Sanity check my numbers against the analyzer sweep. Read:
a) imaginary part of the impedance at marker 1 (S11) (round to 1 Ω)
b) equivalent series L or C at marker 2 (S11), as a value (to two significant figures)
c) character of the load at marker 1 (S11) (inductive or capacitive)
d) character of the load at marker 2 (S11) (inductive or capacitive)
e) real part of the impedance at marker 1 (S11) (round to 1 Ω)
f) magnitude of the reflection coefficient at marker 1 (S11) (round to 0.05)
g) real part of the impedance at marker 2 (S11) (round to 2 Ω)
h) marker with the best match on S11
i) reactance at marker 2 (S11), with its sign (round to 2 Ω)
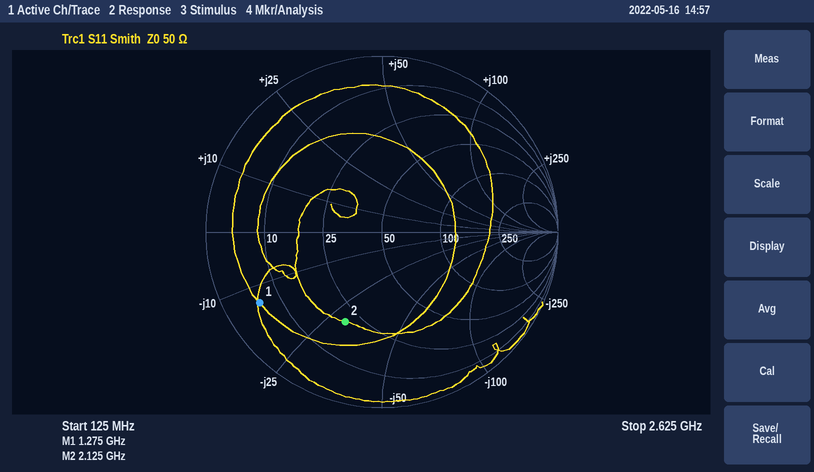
-13 Ω
2.5 pF
capacitive
capacitive
6 Ω
0.80
20 Ω
marker 2
-30 Ω
